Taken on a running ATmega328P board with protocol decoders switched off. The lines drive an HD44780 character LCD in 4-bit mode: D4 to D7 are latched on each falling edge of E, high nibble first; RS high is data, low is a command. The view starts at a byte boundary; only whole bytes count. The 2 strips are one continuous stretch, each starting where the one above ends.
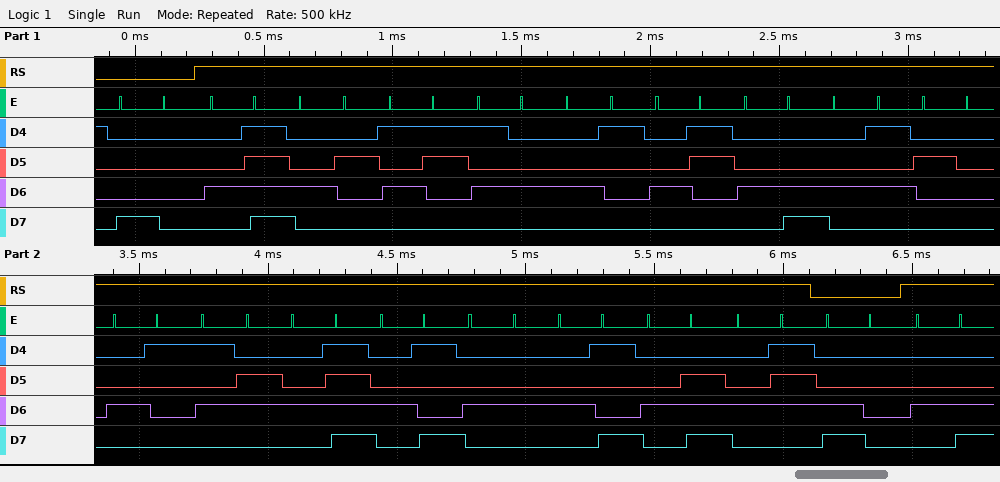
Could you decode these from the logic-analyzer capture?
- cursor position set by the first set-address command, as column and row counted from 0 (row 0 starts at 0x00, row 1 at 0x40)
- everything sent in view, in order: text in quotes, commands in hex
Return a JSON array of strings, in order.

["column 0, row 0", "0x80 \"OBSTACLE AVOIDING\" 0xC0 \"L\""]
